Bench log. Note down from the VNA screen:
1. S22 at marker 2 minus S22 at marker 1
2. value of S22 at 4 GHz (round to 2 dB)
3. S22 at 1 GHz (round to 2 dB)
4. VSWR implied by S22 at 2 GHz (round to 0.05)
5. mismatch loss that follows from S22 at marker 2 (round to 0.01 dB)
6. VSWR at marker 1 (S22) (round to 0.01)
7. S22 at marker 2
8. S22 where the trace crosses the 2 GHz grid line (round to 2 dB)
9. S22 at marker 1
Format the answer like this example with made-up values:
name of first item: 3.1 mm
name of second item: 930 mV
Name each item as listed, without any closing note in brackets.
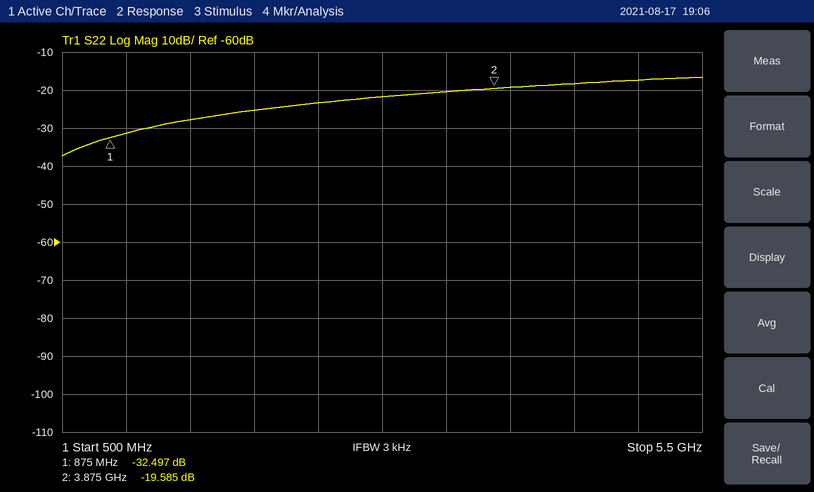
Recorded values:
S22 at marker 2 minus S22 at marker 1: 12.912 dB
value of S22 at 4 GHz: -20 dB
S22 at 1 GHz: -32 dB
VSWR implied by S22 at 2 GHz: 1.10
mismatch loss that follows from S22 at marker 2: 0.05 dB
VSWR at marker 1 (S22): 1.05
S22 at marker 2: -19.585 dB
S22 where the trace crosses the 2 GHz grid line: -26 dB
S22 at marker 1: -32.497 dB
